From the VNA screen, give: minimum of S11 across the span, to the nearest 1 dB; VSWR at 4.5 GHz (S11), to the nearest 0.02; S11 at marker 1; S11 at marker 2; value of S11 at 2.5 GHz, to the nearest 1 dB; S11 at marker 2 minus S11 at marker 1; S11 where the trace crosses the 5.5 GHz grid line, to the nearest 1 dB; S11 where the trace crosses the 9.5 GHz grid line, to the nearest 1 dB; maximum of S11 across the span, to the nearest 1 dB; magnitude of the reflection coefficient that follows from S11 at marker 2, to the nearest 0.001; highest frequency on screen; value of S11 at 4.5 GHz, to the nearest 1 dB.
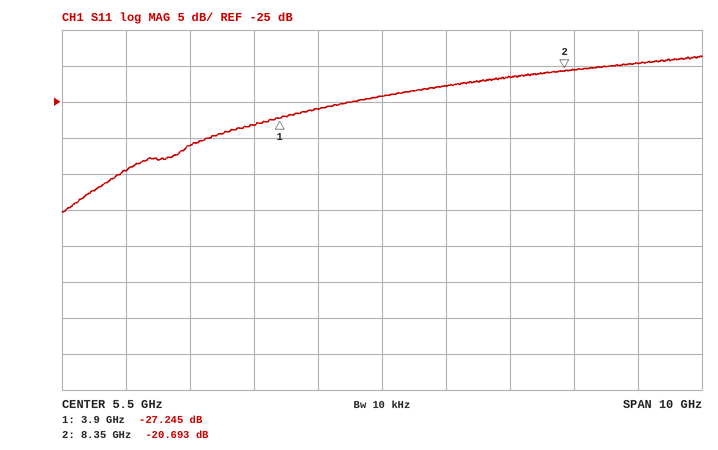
-40 dB
1.10
-27.245 dB
-20.693 dB
-31 dB
6.552 dB
-24 dB
-20 dB
-19 dB
0.092
10.5 GHz
-26 dB
